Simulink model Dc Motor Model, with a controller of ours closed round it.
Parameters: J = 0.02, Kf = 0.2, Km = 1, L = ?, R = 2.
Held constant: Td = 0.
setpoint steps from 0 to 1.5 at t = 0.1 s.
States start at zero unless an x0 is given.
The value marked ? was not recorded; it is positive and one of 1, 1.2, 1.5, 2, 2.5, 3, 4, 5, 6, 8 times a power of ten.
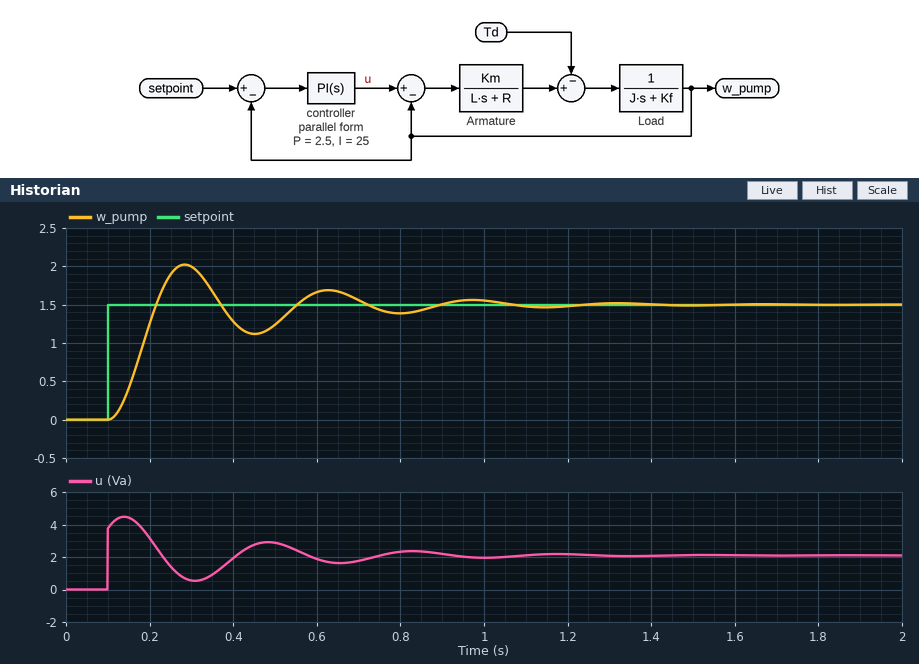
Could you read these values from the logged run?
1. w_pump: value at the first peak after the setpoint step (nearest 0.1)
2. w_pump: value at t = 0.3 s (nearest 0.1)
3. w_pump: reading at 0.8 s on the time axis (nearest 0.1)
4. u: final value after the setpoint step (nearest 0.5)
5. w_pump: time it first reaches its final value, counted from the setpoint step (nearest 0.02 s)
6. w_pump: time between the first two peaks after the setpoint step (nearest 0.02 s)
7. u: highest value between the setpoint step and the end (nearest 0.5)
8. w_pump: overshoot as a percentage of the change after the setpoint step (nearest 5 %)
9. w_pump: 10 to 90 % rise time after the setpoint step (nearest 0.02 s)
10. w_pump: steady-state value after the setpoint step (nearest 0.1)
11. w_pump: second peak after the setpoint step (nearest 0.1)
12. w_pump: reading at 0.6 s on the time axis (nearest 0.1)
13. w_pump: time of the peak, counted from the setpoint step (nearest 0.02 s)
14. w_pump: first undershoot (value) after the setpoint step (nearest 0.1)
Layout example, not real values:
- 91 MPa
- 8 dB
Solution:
- 2.0
- 2.0
- 1.4
- 2.0
- 0.12 s
- 0.34 s
- 4.5
- 35 %
- 0.08 s
- 1.5
- 1.7
- 1.7
- 0.18 s
- 1.1
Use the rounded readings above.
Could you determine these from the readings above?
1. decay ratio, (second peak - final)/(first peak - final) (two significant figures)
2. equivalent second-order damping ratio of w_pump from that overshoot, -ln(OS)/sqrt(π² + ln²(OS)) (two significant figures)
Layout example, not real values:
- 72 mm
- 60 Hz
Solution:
- 0.40
- 0.32
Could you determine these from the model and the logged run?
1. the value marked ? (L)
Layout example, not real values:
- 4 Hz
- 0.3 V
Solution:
- 0.5
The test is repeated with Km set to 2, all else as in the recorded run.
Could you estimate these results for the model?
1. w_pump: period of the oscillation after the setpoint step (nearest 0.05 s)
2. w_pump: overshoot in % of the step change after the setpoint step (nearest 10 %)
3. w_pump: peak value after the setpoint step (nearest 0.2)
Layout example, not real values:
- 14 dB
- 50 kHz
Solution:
- 0.25 s
- 40 %
- 2.0
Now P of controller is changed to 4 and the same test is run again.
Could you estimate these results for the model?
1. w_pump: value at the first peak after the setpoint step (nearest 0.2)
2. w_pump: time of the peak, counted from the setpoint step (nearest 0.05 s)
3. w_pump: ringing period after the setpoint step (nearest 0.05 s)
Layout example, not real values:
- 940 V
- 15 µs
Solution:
- 2.0
- 0.15 s
- 0.30 s
